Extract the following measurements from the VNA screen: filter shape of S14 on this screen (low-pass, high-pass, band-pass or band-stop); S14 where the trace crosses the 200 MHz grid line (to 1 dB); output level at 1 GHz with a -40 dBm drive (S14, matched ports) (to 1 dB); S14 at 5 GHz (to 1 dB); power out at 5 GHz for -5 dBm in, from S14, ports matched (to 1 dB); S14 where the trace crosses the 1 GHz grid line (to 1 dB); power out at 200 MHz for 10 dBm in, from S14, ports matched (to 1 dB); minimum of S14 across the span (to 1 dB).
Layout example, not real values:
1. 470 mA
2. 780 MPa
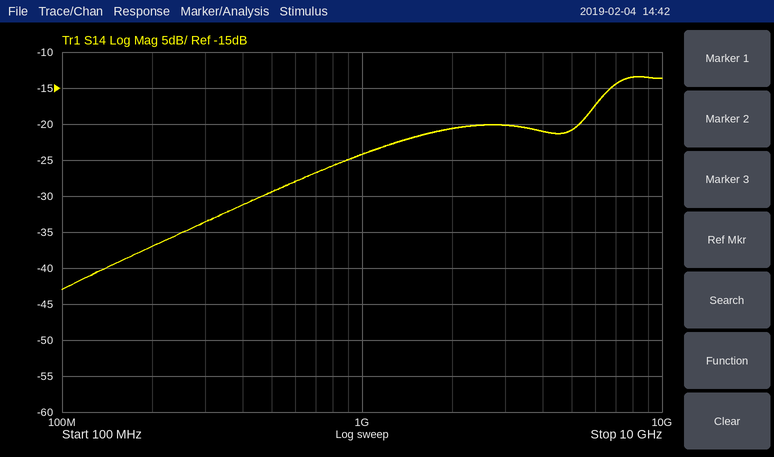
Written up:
1. high-pass
2. -37 dB
3. -64 dBm
4. -21 dB
5. -26 dBm
6. -24 dB
7. -27 dBm
8. -43 dB
